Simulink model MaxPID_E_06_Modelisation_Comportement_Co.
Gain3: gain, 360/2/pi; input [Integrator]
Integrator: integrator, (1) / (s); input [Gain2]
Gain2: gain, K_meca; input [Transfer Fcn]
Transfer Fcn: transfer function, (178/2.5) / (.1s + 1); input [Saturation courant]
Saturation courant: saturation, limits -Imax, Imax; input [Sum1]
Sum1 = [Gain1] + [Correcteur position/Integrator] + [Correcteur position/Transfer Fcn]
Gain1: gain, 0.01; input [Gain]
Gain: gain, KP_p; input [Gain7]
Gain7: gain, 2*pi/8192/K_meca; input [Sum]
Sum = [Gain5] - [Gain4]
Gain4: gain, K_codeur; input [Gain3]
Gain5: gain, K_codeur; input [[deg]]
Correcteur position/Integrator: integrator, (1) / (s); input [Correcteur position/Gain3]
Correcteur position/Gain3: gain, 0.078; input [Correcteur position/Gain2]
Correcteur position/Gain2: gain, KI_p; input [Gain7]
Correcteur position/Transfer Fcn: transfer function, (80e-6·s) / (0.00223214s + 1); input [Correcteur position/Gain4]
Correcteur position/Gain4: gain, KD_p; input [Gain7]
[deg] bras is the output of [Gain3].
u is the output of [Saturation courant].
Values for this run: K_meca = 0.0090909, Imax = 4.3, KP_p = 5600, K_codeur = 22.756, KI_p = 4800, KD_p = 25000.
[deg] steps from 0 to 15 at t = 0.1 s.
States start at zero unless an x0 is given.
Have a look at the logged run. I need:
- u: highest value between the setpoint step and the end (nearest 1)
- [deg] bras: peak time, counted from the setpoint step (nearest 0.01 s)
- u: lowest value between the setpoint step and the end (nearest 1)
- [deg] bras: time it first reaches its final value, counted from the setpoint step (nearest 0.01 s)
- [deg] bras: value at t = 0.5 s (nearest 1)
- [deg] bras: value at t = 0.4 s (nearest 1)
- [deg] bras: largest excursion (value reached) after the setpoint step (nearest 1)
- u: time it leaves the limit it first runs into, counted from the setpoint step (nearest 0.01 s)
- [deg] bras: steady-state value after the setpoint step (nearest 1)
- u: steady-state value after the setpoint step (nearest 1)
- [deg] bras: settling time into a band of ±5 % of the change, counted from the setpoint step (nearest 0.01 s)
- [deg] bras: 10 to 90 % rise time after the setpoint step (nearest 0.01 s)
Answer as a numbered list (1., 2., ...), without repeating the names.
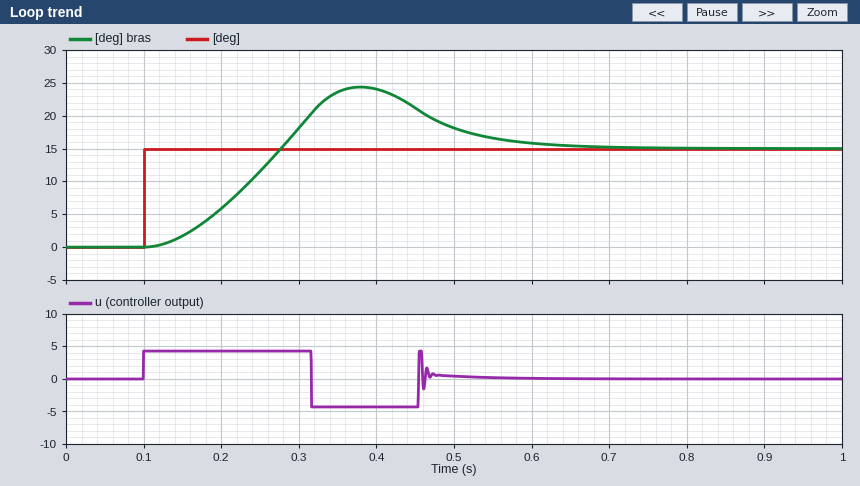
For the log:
1. 4
2. 0.28 s
3. -4
4. 0.18 s
5. 18
6. 24
7. 24
8. 0.22 s
9. 15
10. 0
11. 0.51 s
12. 0.12 s
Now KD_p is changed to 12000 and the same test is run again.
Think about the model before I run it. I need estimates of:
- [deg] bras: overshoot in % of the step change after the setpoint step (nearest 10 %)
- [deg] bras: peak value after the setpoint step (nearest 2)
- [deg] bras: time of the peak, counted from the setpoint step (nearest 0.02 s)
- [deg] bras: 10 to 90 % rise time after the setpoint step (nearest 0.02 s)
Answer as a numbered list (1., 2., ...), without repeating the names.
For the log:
1. 80 %
2. 26
3. 0.30 s
4. 0.12 s
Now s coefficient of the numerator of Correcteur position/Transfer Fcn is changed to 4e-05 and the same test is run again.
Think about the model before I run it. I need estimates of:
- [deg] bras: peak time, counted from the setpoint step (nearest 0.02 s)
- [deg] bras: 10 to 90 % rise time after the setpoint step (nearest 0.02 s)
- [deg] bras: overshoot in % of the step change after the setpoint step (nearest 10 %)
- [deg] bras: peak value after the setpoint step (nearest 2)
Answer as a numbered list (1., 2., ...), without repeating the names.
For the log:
1. 0.30 s
2. 0.12 s
3. 80 %
4. 26
